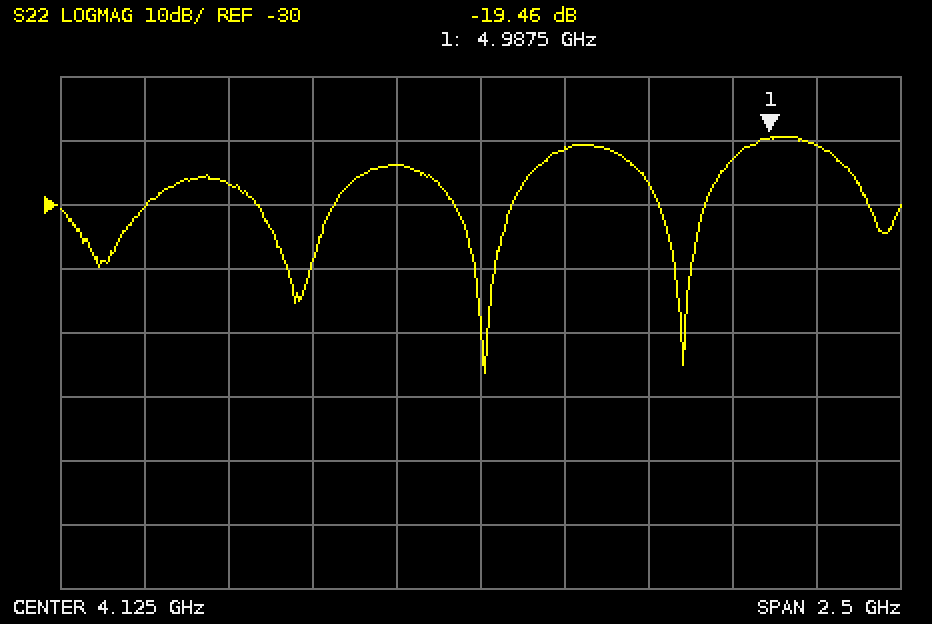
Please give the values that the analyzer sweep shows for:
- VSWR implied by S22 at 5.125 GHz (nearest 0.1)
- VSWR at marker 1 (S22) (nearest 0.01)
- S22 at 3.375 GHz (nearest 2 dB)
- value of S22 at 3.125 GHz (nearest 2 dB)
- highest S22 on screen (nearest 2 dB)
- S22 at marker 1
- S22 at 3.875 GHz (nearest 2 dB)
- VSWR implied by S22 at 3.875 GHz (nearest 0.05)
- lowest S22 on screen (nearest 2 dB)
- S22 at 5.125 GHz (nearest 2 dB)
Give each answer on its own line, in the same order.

1.2
1.24
-26 dB
-30 dB
-20 dB
-19.46 dB
-24 dB
1.15
-56 dB
-20 dB
